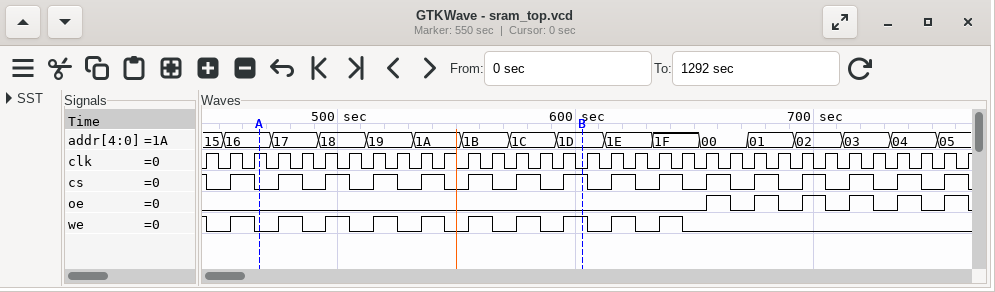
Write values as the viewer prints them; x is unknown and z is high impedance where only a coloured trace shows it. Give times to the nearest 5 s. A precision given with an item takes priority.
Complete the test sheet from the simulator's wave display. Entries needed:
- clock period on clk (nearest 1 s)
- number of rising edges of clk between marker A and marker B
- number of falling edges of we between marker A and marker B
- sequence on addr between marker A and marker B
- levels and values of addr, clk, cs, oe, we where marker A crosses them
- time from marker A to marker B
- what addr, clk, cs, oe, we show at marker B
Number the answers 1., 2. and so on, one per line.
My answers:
1. 10 s
2. 13
3. 6
4. 16, 17, 18, 19, 1A, 1B, 1C, 1D
5. addr=16, clk=1, cs=0, oe=0, we=0
6. 135 s
7. addr=1D, clk=0, cs=1, oe=0, we=1
